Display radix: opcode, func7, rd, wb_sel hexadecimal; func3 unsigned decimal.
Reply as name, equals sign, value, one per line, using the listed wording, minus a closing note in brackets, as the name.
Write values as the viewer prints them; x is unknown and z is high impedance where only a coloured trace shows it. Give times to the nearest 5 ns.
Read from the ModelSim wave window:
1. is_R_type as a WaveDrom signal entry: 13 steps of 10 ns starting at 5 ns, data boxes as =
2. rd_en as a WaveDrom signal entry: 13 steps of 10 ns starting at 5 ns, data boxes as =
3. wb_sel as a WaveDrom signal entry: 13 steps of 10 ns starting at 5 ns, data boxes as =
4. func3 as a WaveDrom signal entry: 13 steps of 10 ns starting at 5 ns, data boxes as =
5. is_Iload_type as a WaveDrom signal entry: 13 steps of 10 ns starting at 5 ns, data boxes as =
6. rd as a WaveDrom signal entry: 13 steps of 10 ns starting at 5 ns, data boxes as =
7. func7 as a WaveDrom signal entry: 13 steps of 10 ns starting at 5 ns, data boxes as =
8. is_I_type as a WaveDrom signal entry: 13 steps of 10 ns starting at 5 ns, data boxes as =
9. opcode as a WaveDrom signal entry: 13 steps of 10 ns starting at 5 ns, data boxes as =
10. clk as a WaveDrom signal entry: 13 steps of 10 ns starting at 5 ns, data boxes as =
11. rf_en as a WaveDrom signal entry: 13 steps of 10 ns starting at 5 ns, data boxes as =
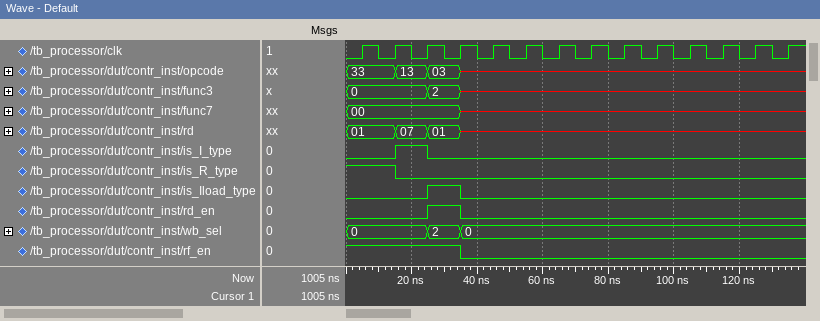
is_R_type as a WaveDrom signal entry: 13 steps of 10 ns starting at 5 ns, data boxes as = = {name: 'is_R_type', wave: '10...........'}
rd_en as a WaveDrom signal entry: 13 steps of 10 ns starting at 5 ns, data boxes as = = {name: 'rd_en', wave: '0.10.........'}
wb_sel as a WaveDrom signal entry: 13 steps of 10 ns starting at 5 ns, data boxes as = = {name: 'wb_sel', wave: '=.==.........', data: '0 2 0'}
func3 as a WaveDrom signal entry: 13 steps of 10 ns starting at 5 ns, data boxes as = = {name: 'func3', wave: '=.=x.........', data: '0 2'}
is_Iload_type as a WaveDrom signal entry: 13 steps of 10 ns starting at 5 ns, data boxes as = = {name: 'is_Iload_type', wave: '0.10.........'}
rd as a WaveDrom signal entry: 13 steps of 10 ns starting at 5 ns, data boxes as = = {name: 'rd', wave: '===x.........', data: '01 07 01'}
func7 as a WaveDrom signal entry: 13 steps of 10 ns starting at 5 ns, data boxes as = = {name: 'func7', wave: '=..x.........', data: '00'}
is_I_type as a WaveDrom signal entry: 13 steps of 10 ns starting at 5 ns, data boxes as = = {name: 'is_I_type', wave: '010..........'}
opcode as a WaveDrom signal entry: 13 steps of 10 ns starting at 5 ns, data boxes as = = {name: 'opcode', wave: '===x.........', data: '33 13 03'}
clk as a WaveDrom signal entry: 13 steps of 10 ns starting at 5 ns, data boxes as = = {name: 'clk', wave: 'p............'}
rf_en as a WaveDrom signal entry: 13 steps of 10 ns starting at 5 ns, data boxes as = = {name: 'rf_en', wave: '1..0.........'}
